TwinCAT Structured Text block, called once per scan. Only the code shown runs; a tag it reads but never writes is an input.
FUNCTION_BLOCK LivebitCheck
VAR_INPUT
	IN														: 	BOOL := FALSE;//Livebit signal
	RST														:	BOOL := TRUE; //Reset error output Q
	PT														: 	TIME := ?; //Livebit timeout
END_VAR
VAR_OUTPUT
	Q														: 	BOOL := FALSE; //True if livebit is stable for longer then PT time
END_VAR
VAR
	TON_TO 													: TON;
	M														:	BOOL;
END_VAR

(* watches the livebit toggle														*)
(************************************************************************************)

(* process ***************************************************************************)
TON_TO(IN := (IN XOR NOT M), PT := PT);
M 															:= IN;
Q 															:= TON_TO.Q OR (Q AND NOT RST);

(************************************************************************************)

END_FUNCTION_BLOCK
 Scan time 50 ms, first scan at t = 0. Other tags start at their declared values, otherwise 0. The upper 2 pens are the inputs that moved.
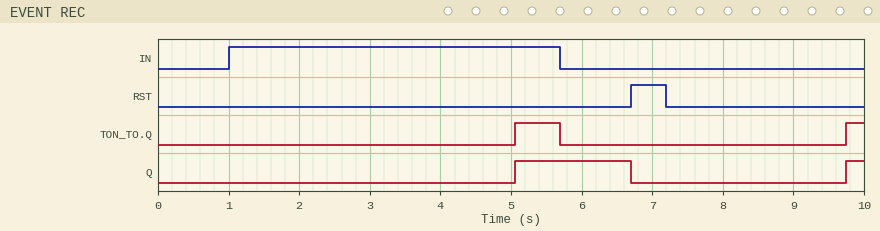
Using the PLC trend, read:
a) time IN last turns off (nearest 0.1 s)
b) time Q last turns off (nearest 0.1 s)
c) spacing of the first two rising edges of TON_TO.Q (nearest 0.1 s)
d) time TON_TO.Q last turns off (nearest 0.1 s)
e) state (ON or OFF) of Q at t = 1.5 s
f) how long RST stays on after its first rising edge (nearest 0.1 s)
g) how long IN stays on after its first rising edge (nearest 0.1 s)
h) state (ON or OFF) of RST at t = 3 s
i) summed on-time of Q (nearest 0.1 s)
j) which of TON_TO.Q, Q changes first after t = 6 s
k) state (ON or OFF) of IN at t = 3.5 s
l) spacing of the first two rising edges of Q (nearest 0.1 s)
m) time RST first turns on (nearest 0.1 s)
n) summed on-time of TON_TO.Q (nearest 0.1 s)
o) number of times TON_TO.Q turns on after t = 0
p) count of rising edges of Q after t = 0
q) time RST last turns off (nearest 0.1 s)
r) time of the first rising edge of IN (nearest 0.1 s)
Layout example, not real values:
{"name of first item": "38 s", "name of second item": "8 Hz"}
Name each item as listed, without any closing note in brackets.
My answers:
{"time IN last turns off": "5.7 s", "time Q last turns off": "6.7 s", "spacing of the first two rising edges of TON_TO.Q": "4.7 s", "time TON_TO.Q last turns off": "5.7 s", "state (ON or OFF) of Q at t = 1.5 s": "OFF", "how long RST stays on after its first rising edge": "0.5 s", "how long IN stays on after its first rising edge": "4.7 s", "state (ON or OFF) of RST at t = 3 s": "OFF", "summed on-time of Q": "1.9 s", "which of TON_TO.Q, Q changes first after t = 6 s": "Q", "state (ON or OFF) of IN at t = 3.5 s": "ON", "spacing of the first two rising edges of Q": "4.7 s", "time RST first turns on": "6.7 s", "summed on-time of TON_TO.Q": "0.9 s", "number of times TON_TO.Q turns on after t = 0": "2", "count of rising edges of Q after t = 0": "2", "time RST last turns off": "7.2 s", "time of the first rising edge of IN": "1.0 s"}
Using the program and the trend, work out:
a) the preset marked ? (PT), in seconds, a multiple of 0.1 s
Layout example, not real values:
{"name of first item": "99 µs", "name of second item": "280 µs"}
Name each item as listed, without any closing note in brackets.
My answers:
{"the preset marked ? (PT), in seconds, a multiple of 0.1 s": "4.0 s"}
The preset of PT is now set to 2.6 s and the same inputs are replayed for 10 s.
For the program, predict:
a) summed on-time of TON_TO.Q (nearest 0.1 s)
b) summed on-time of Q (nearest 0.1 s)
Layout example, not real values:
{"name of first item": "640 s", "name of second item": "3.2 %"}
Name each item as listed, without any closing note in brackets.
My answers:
{"summed on-time of TON_TO.Q": "3.7 s", "summed on-time of Q": "4.7 s"}
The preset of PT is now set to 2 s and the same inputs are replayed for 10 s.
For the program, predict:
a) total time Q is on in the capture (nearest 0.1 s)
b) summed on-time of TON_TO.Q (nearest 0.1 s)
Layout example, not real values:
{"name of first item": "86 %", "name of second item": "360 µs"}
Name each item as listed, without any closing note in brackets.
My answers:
{"total time Q is on in the capture": "5.9 s", "summed on-time of TON_TO.Q": "4.9 s"}
